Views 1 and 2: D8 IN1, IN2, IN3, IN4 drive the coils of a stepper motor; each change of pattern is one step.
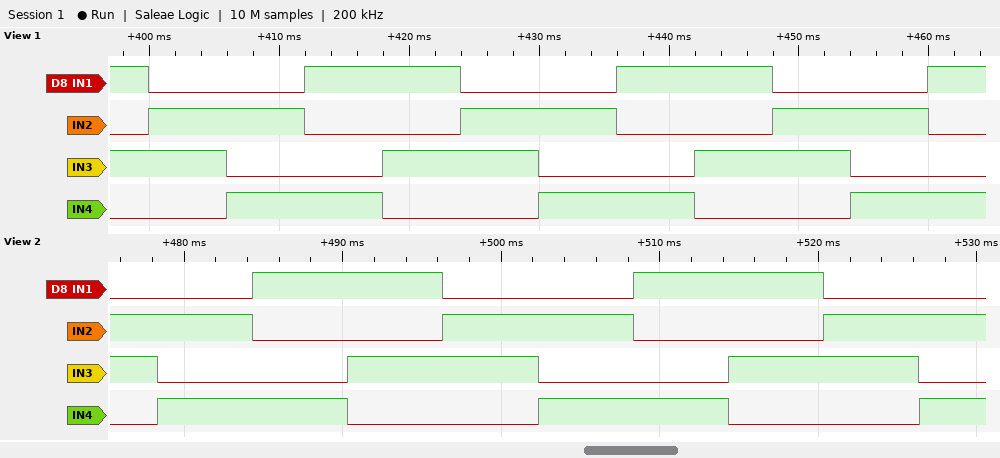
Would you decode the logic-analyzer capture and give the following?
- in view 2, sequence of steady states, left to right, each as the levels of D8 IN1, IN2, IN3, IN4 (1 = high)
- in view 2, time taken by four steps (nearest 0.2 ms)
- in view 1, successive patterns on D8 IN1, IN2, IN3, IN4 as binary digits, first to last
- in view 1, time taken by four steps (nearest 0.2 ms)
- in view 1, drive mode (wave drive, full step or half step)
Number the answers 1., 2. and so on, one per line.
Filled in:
1. 0110 0101 1001 1010 0110 0101 1001 1010 0110 0101
2. 24.0 ms
3. 1010 0110 0101 1001 1010 0110 0101 1001 1010 0110 0101 1001
4. 24.0 ms
5. full step
